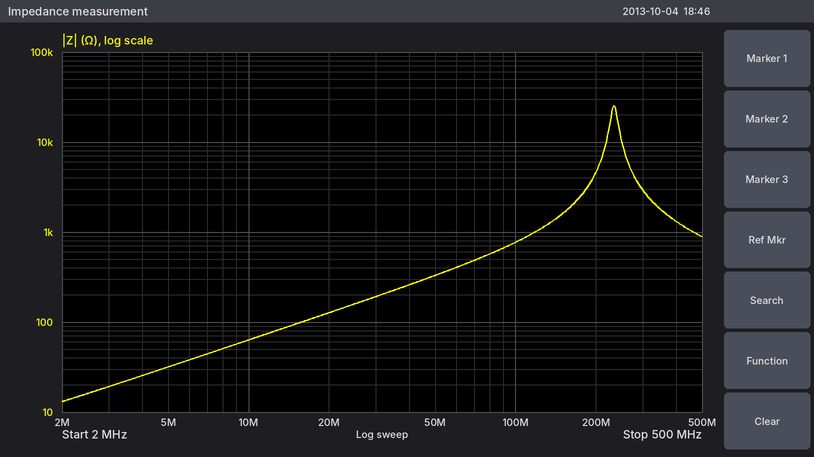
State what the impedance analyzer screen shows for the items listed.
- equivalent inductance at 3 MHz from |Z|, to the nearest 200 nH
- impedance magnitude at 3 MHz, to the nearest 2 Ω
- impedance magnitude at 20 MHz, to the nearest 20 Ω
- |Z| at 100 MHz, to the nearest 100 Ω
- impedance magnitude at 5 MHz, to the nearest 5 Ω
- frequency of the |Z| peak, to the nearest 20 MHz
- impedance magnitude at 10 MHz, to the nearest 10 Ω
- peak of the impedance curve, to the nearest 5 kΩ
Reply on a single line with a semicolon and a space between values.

1.0 µH; 20 Ω; 120 Ω; 800 Ω; 30 Ω; 240 MHz; 60 Ω; 25 kΩ
